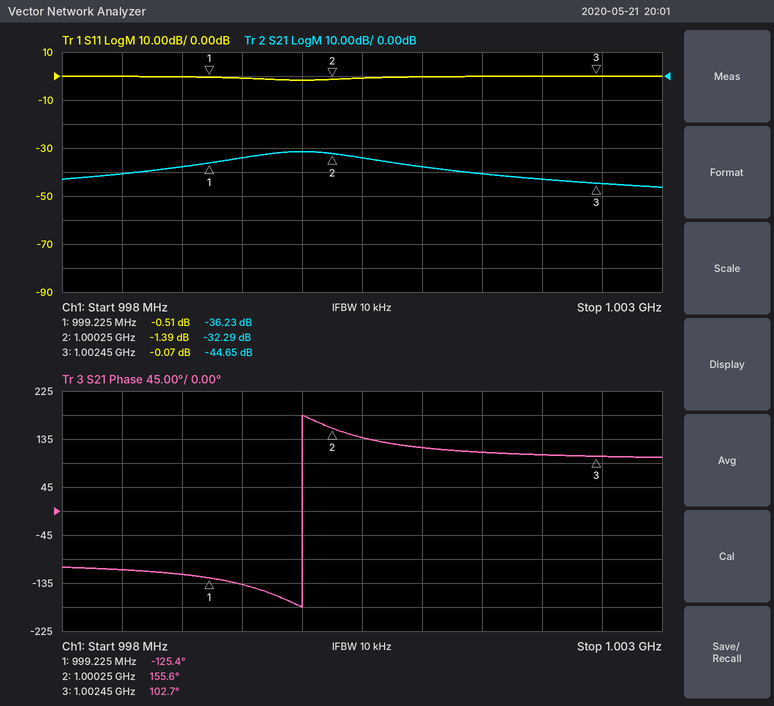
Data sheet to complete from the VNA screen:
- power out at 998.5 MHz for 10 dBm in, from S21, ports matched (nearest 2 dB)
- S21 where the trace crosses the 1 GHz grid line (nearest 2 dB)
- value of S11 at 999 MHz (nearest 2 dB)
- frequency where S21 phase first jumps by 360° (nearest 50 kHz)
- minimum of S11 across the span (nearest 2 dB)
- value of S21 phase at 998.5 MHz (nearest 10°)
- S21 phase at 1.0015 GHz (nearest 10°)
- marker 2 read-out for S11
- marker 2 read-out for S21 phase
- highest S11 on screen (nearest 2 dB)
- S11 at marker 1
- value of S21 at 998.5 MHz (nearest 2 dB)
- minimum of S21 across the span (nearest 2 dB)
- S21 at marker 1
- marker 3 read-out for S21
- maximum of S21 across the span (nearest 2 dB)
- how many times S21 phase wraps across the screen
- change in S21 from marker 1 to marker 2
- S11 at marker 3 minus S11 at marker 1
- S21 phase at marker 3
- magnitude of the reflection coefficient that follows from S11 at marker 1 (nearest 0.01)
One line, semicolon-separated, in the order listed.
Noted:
-30 dBm; -32 dB; 0 dB; 1.00000 GHz; -2 dB; -110°; 110°; -1.39 dB; 155.6°; 0 dB; -0.51 dB; -40 dB; -46 dB; -36.23 dB; -44.65 dB; -32 dB; 1; 3.94 dB; 0.44 dB; 102.7°; 0.94
